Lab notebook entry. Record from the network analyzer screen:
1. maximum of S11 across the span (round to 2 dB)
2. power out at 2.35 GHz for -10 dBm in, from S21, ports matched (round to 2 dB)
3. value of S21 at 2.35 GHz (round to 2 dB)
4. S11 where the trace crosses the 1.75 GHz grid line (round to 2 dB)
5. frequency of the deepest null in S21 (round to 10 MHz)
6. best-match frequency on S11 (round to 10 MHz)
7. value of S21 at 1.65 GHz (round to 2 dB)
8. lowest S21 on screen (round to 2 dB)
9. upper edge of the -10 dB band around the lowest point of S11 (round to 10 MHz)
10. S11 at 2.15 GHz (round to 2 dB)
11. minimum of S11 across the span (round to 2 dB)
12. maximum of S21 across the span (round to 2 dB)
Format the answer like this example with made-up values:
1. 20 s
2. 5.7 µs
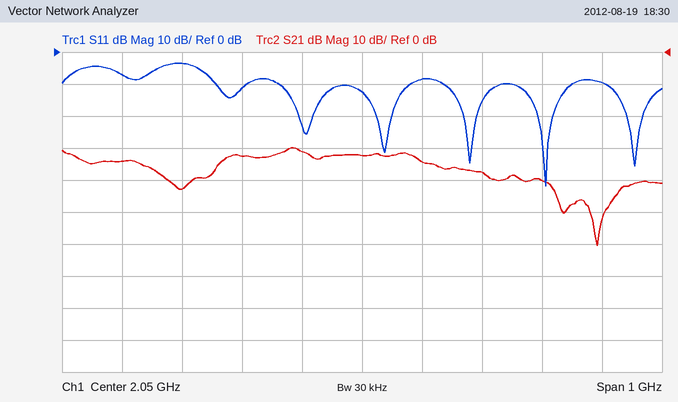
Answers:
1. -4 dB
2. -50 dBm
3. -40 dB
4. -4 dB
5. 2.44 GHz
6. 2.36 GHz
7. -34 dB
8. -60 dB
9. 2.40 GHz
10. -8 dB
11. -42 dB
12. -30 dB
